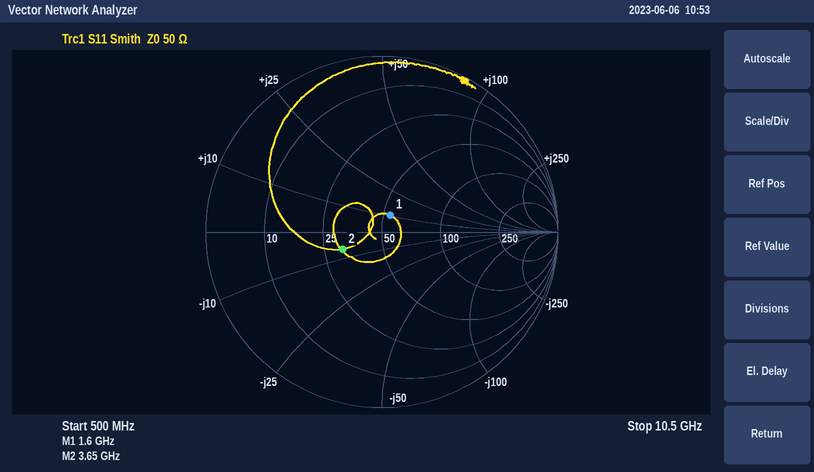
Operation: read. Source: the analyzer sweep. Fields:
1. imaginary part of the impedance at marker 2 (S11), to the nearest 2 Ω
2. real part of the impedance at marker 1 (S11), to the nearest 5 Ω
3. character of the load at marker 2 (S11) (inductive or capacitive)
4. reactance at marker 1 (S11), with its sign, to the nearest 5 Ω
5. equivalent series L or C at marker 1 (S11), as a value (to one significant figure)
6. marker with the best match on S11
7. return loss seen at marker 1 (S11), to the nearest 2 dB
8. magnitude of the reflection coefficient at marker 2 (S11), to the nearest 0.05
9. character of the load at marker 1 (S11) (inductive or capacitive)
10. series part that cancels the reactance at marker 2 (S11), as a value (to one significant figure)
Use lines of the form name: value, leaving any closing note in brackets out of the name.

imaginary part of the impedance at marker 2 (S11), to the nearest 2 Ω: -6 Ω
real part of the impedance at marker 1 (S11), to the nearest 5 Ω: 55 Ω
character of the load at marker 2 (S11): capacitive
reactance at marker 1 (S11), with its sign, to the nearest 5 Ω: +10 Ω
equivalent series L or C at marker 1 (S11), as a value: 1 nH
marker with the best match on S11: marker 1
return loss seen at marker 1 (S11), to the nearest 2 dB: 20 dB
magnitude of the reflection coefficient at marker 2 (S11), to the nearest 0.05: 0.25
character of the load at marker 1 (S11): inductive
series part that cancels the reactance at marker 2 (S11), as a value: 300 pH
